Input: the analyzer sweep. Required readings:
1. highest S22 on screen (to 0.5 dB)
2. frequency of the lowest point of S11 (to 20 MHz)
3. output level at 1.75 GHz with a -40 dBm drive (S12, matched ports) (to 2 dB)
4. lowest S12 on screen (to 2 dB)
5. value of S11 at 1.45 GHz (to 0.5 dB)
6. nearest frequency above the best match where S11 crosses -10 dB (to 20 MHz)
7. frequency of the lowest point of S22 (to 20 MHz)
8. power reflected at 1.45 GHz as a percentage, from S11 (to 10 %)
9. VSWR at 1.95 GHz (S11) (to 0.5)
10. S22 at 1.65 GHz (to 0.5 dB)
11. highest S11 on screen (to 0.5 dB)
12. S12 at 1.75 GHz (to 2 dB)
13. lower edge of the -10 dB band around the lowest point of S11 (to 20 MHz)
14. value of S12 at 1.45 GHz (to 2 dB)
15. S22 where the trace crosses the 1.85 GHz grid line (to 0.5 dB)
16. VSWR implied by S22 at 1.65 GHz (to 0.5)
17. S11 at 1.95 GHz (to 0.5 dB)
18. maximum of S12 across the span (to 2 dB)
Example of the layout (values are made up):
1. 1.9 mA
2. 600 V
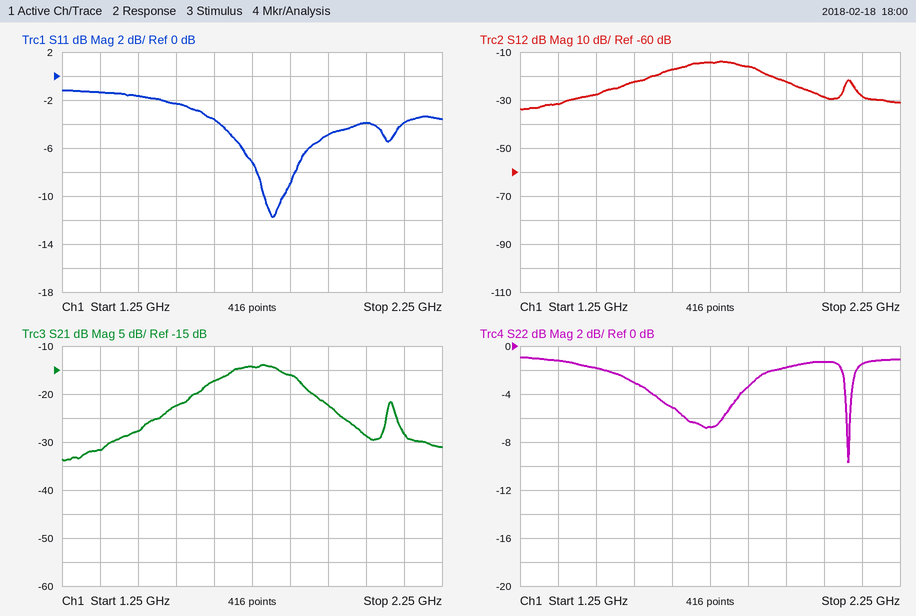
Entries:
1. -1.0 dB
2. 1.80 GHz
3. -54 dBm
4. -34 dB
5. -1.5 dB
6. 1.84 GHz
7. 2.12 GHz
8. 70 %
9. 3.5
10. -5.0 dB
11. -1.0 dB
12. -14 dB
13. 1.78 GHz
14. -28 dB
15. -3.5 dB
16. 3.5
17. -5.0 dB
18. -14 dB
